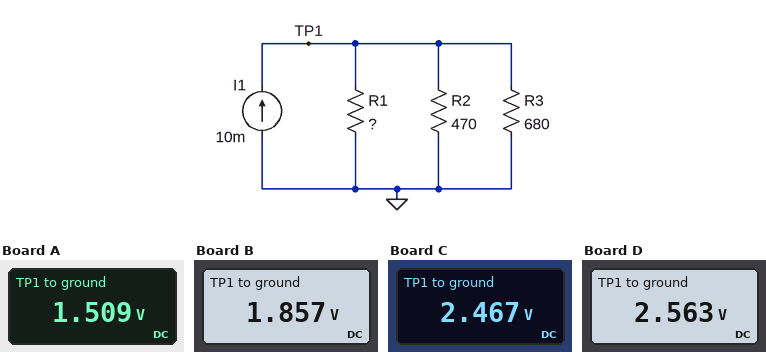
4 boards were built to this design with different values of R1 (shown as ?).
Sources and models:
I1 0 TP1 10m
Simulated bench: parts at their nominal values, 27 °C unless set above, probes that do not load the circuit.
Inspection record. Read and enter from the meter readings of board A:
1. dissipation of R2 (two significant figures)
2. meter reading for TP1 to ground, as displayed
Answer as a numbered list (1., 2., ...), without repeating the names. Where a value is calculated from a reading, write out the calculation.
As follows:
1. (1.509 V)^2 / 470 Ω = 4.8 mW
2. 1.509 V
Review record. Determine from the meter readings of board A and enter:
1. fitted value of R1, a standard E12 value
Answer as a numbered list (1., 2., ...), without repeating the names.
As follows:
1. 330 Ω
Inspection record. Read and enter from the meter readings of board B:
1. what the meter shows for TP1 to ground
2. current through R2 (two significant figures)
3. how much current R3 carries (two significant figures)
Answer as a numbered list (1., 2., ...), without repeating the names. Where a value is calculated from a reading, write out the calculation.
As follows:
1. 1.857 V
2. (1.857 V) / 470 Ω = 4.0 mA
3. (1.857 V) / 680 Ω = 2.7 mA
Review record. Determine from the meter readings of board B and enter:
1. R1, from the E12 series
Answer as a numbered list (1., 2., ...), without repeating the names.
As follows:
1. 560 Ω
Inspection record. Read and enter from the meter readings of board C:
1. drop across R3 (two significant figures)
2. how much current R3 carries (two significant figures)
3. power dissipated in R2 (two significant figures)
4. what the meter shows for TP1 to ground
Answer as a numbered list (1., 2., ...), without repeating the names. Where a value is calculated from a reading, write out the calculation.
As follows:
1. 2.467 V = 2.5 V
2. (2.467 V) / 680 Ω = 3.6 mA
3. (2.467 V)^2 / 470 Ω = 13 mW
4. 2.467 V
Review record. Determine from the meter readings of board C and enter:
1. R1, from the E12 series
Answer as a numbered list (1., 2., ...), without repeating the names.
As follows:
1. 2.2 kΩ
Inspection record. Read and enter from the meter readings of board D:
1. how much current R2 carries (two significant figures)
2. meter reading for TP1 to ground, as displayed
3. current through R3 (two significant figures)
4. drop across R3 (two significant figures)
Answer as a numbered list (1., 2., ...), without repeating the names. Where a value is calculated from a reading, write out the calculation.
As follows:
1. (2.563 V) / 470 Ω = 5.5 mA
2. 2.563 V
3. (2.563 V) / 680 Ω = 3.8 mA
4. 2.563 V = 2.6 V
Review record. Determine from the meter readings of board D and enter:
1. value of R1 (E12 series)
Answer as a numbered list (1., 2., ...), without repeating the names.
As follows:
1. 3.3 kΩ
